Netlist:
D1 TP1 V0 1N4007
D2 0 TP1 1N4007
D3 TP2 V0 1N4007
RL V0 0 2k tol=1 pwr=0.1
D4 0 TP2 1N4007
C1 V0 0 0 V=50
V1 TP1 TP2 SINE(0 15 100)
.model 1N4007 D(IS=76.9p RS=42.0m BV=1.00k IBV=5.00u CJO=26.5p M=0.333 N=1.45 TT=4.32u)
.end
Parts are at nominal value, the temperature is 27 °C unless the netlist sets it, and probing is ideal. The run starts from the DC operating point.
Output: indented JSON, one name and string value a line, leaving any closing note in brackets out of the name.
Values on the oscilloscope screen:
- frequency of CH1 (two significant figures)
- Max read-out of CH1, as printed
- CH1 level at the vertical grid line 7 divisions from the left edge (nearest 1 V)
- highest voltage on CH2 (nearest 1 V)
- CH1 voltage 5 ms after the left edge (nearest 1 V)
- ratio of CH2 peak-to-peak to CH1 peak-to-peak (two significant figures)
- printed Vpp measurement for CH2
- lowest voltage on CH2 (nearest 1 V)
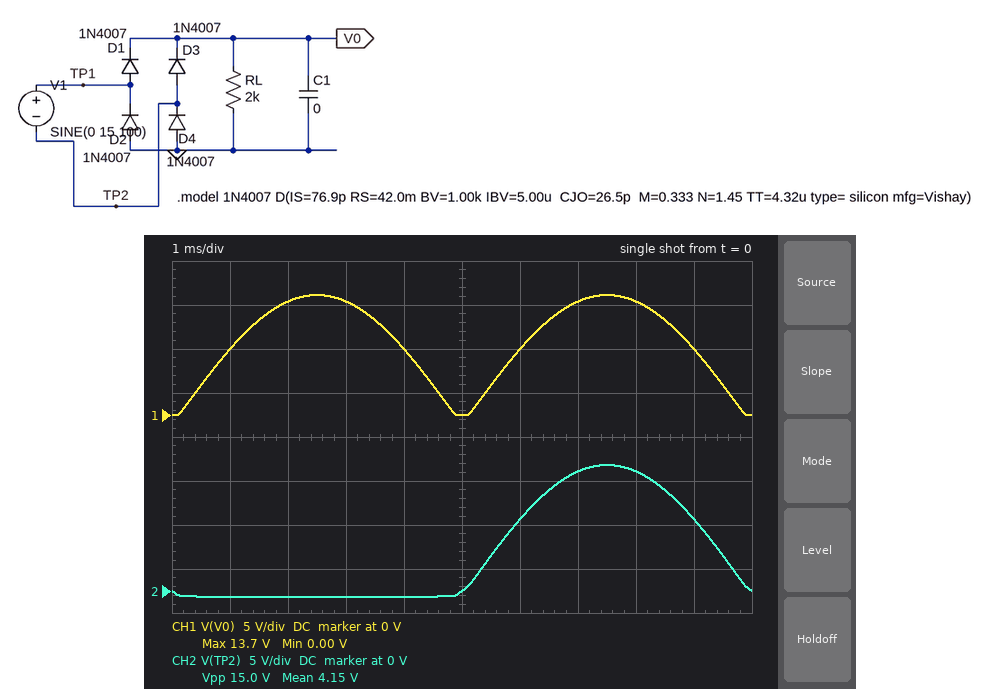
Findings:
{
  "frequency of CH1": "200 Hz",
  "Max read-out of CH1, as printed": "13.7 V",
  "CH1 level at the vertical grid line 7 divisions from the left edge": "13 V",
  "highest voltage on CH2": "14 V",
  "CH1 voltage 5 ms after the left edge": "0 V",
  "ratio of CH2 peak-to-peak to CH1 peak-to-peak": "1.1",
  "printed Vpp measurement for CH2": "15.0 V",
  "lowest voltage on CH2": "-1 V"
}
